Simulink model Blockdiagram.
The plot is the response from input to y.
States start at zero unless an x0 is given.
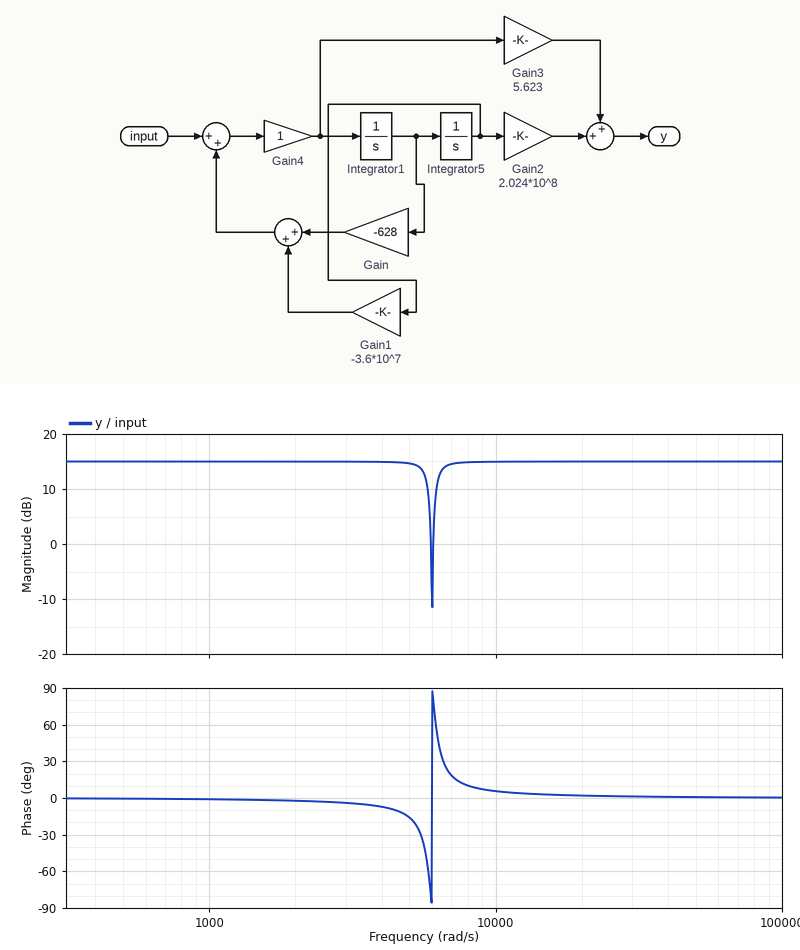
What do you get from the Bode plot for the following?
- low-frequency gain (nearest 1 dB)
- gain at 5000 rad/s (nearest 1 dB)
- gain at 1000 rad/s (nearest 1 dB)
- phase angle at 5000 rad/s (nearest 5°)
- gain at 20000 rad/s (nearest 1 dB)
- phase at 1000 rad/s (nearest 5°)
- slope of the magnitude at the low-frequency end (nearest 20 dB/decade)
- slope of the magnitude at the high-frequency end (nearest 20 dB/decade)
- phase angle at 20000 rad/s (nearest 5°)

15 dB
15 dB
15 dB
-15°
15 dB
0°
0 dB/decade
0 dB/decade
0°
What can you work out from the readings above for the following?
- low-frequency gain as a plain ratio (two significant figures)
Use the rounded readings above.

5.6
